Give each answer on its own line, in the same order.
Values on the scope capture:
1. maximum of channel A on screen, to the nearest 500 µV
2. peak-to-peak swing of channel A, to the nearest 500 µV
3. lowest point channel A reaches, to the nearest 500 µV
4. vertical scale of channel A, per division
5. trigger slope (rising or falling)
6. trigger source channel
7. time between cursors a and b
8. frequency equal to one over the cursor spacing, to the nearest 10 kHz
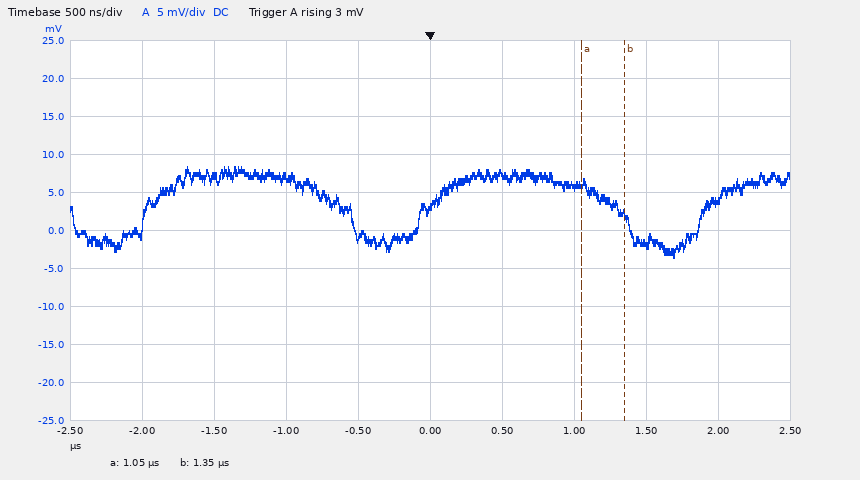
8.5 mV
12.0 mV
-3.5 mV
5 mV
rising
channel A
300 ns
3.33 MHz
